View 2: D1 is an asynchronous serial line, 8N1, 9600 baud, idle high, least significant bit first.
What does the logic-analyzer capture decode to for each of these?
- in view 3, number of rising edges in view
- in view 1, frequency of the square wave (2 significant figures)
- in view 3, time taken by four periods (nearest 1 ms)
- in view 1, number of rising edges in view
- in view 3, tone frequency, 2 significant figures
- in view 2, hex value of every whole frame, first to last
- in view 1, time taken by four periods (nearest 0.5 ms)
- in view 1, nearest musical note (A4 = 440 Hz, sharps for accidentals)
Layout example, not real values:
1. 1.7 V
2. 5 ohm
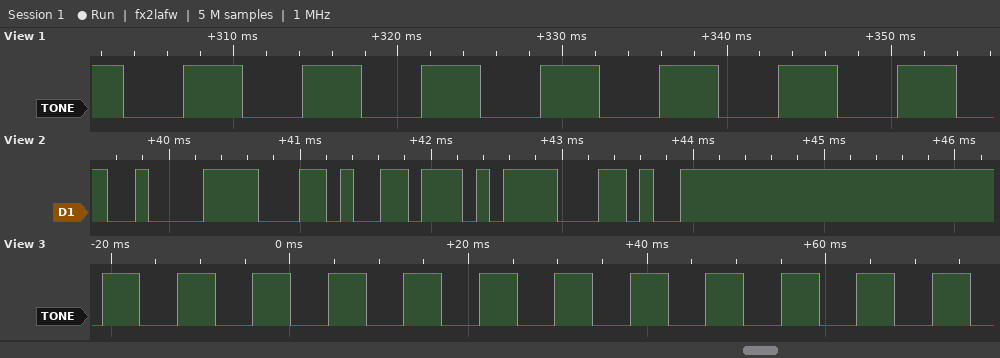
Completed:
1. 12
2. 140 Hz
3. 34 ms
4. 7
5. 120 Hz
6. C2 2C D7 2C
7. 29.0 ms
8. C#3
